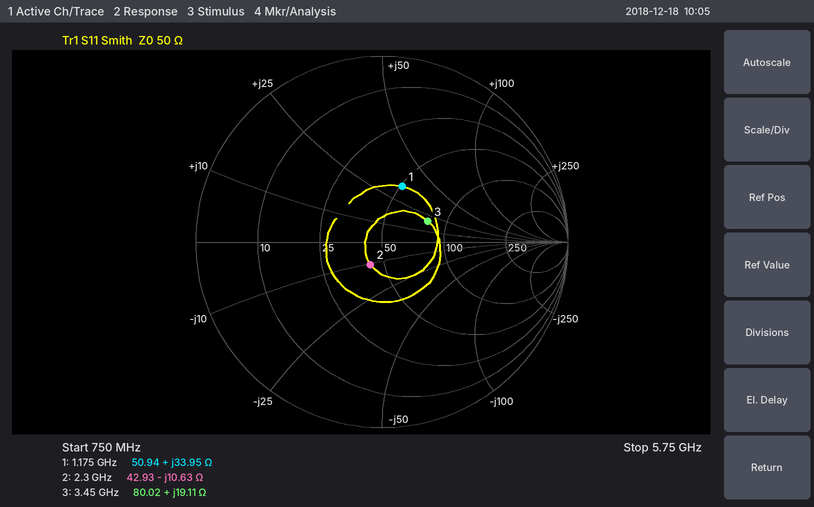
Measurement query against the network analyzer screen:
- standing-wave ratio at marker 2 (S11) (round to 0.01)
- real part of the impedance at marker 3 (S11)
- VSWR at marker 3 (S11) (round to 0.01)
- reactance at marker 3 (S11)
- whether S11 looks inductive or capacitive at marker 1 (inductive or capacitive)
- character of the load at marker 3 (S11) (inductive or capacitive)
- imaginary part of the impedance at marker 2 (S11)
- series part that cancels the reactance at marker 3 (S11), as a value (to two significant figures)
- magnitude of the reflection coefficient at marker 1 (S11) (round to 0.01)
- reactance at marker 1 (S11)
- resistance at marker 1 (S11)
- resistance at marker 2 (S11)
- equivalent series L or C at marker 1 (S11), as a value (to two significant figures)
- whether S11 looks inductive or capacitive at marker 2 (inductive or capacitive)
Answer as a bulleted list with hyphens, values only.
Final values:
- 1.32
- 80.02 Ω
- 1.74
- +19.11 Ω
- inductive
- inductive
- -10.63 Ω
- 2.4 pF
- 0.32
- +33.95 Ω
- 50.94 Ω
- 42.93 Ω
- 4.6 nH
- capacitive
